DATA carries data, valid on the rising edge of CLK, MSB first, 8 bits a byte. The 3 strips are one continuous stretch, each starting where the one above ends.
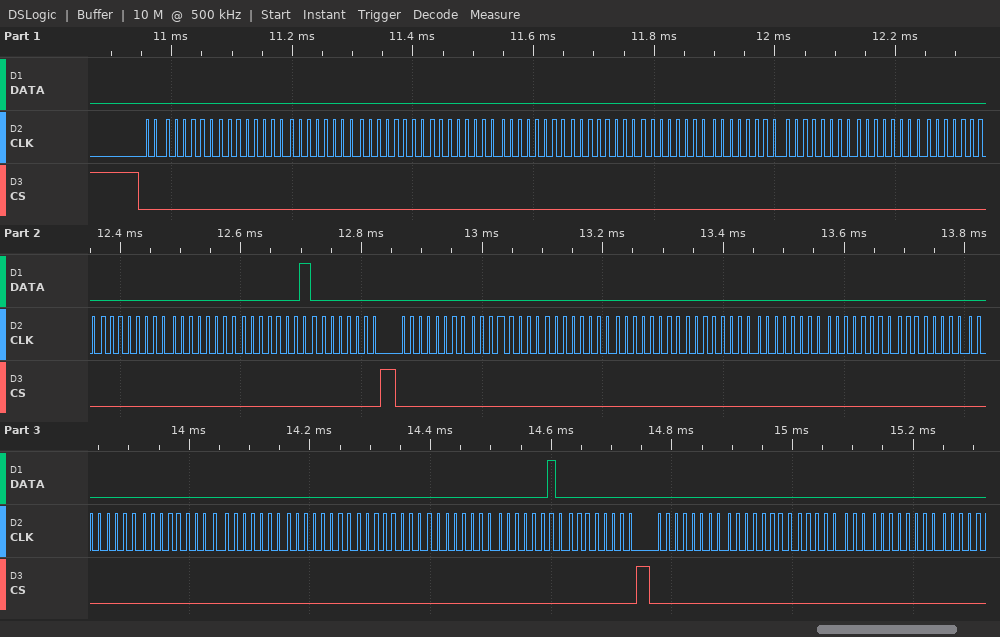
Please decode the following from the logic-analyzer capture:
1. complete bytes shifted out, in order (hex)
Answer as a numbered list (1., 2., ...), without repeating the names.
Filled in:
1. 00 00 00 00 00 00 00 00 00 00 00 00 00 00 01 00 00 00 00 00 00 00 00 00 00 00 00 00 00 00 02 00 00 00 00 00
